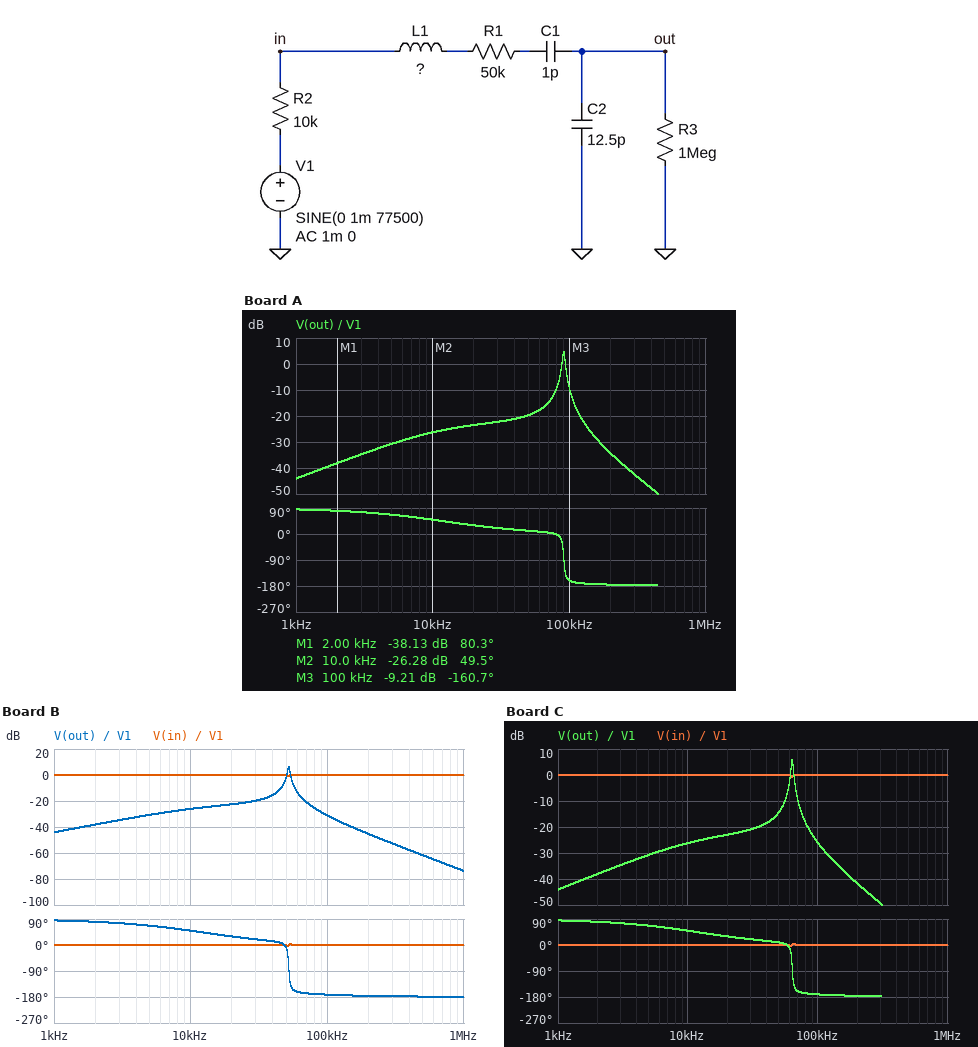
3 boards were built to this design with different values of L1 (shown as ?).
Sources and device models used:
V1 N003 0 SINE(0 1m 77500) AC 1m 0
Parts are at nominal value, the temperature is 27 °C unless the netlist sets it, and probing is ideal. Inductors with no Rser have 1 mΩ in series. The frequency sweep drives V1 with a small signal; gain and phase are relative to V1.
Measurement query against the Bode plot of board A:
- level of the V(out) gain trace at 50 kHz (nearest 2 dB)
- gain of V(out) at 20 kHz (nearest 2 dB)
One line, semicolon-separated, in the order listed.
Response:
-20 dB; -24 dB
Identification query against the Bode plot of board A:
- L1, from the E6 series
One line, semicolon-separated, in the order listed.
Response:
3.3 H
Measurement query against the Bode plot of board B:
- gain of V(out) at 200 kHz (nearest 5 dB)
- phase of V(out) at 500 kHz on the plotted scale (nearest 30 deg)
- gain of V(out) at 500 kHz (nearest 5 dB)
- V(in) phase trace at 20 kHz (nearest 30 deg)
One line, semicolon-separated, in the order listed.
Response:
-45 dB; -180 deg; -60 dB; 0 deg
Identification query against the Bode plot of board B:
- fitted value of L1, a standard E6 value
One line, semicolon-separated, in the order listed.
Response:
10 H
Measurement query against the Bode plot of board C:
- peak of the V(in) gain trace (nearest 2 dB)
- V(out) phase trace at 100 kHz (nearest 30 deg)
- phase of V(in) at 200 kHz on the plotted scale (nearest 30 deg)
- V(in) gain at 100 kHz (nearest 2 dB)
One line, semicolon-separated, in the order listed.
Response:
0 dB; -180 deg; 0 deg; 0 dB
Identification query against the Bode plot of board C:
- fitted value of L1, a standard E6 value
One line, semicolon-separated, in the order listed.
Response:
6.8 H
